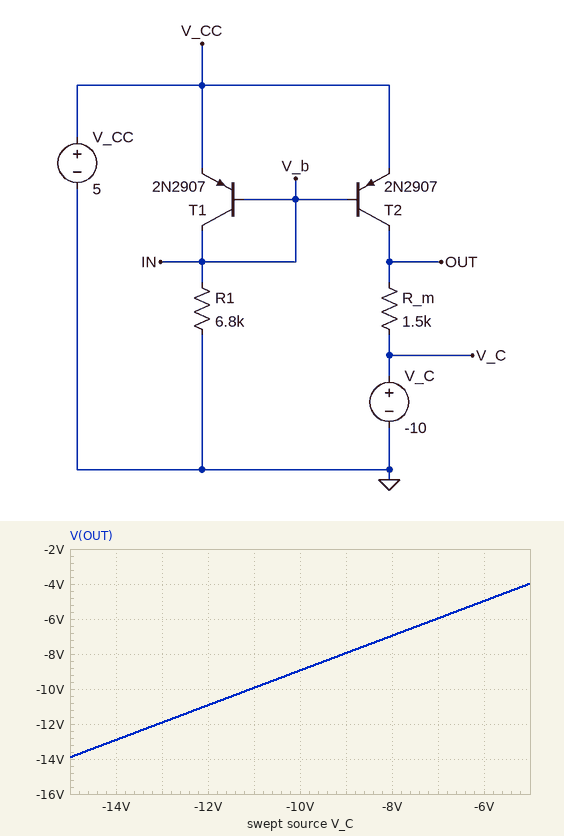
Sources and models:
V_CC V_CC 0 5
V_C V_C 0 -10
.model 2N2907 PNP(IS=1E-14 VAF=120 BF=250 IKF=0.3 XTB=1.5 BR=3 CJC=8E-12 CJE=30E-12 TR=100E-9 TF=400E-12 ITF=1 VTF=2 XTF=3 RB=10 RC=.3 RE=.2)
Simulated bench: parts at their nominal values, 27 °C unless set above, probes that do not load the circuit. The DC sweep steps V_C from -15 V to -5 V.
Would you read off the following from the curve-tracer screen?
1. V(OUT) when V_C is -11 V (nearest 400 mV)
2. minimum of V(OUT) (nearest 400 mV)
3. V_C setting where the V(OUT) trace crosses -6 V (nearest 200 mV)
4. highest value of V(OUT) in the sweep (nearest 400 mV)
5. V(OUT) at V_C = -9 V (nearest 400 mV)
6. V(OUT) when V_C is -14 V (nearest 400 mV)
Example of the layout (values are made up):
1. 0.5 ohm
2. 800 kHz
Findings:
1. -10.0 V
2. -14.0 V
3. -7.0 V
4. -4.0 V
5. -8.0 V
6. -12.8 V
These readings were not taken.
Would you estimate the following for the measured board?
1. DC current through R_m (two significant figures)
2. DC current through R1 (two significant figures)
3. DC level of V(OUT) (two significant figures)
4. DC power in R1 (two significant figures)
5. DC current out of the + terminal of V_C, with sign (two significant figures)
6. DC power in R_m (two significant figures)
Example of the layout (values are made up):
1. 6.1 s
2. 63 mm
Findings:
1. 710 µA
2. 640 µA
3. -8.9 V
4. 2.8 mW
5. -710 µA
6. 750 µW
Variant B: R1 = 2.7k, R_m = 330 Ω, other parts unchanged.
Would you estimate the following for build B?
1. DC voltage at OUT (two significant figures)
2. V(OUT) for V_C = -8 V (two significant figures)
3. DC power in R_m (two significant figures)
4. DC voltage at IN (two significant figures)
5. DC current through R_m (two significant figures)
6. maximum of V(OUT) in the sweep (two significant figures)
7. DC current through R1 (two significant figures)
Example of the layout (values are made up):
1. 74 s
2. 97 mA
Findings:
1. -9.4 V
2. -7.4 V
3. 1.0 mW
4. 4.3 V
5. 1.8 mA
6. -4.4 V
7. 1.6 mA
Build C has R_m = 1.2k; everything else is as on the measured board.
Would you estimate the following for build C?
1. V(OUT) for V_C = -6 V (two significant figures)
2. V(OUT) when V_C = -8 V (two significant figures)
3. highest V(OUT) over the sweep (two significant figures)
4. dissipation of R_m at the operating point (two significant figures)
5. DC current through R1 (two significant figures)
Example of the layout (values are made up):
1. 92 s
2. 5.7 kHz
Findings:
1. -5.2 V
2. -7.2 V
3. -4.2 V
4. 600 µW
5. 640 µA
